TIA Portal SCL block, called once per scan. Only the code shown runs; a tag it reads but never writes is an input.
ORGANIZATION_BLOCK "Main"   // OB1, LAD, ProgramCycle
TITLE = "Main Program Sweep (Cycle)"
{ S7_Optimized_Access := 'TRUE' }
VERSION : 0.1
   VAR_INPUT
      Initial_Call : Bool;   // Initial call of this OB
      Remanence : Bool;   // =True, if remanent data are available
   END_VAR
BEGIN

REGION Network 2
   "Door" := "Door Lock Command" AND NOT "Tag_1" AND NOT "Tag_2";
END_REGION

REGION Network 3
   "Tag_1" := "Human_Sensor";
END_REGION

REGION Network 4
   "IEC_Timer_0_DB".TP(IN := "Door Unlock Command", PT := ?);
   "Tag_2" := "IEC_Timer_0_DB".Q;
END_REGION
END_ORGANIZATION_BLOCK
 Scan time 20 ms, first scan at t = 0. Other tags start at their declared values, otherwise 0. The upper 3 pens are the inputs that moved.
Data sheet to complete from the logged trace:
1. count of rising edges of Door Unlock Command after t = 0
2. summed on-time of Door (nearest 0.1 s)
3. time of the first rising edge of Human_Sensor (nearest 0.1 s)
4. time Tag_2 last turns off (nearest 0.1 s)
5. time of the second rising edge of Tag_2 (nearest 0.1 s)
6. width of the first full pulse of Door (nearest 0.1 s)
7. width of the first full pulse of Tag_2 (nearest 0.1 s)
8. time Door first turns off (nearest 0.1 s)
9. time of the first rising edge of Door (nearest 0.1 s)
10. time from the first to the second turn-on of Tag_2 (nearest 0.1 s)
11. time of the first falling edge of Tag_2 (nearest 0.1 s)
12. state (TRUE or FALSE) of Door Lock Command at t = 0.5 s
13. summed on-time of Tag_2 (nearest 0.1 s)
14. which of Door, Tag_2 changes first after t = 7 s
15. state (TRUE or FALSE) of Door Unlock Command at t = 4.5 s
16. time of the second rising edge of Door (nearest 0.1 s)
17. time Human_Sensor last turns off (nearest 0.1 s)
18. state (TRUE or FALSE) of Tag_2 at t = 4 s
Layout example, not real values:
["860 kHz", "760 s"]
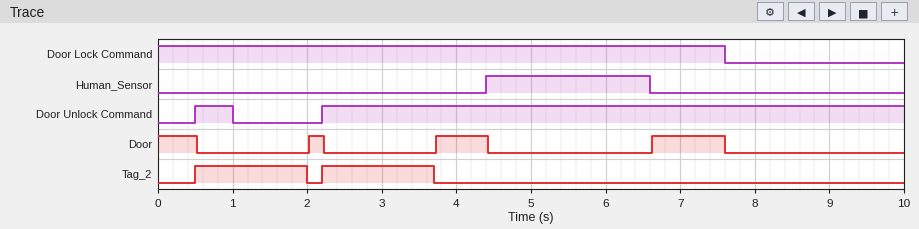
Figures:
["2", "2.4 s", "4.4 s", "3.7 s", "2.2 s", "0.2 s", "1.5 s", "0.5 s", "2.0 s", "1.7 s", "2.0 s", "TRUE", "3.0 s", "Door", "TRUE", "3.7 s", "6.6 s", "FALSE"]
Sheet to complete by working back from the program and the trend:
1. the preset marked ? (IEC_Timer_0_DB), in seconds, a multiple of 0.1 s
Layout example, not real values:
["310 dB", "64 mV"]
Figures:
["1.5 s"]
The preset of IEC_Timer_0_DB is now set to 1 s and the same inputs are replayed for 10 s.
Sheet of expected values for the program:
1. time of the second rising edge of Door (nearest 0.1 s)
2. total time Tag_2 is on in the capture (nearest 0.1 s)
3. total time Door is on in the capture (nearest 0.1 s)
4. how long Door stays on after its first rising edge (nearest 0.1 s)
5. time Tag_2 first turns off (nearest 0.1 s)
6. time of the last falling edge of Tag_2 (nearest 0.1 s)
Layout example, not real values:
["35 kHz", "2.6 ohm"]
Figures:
["3.2 s", "2.0 s", "3.4 s", "0.7 s", "1.5 s", "3.2 s"]
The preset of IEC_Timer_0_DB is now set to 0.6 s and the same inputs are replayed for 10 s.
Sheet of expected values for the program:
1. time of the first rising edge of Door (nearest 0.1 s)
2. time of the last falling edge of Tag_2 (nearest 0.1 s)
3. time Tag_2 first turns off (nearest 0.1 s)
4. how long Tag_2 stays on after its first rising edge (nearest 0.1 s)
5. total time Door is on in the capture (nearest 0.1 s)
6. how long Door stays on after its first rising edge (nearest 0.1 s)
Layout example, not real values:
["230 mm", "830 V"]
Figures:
["1.1 s", "2.8 s", "1.1 s", "0.6 s", "4.2 s", "1.1 s"]
